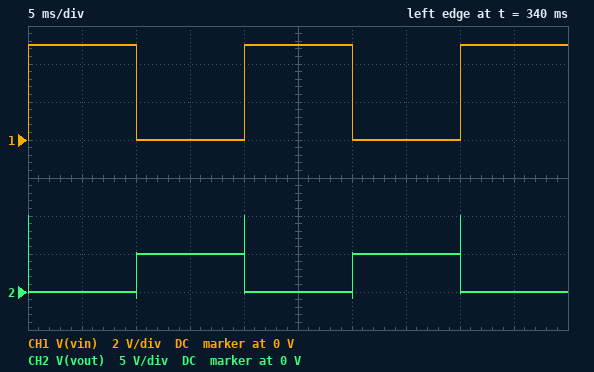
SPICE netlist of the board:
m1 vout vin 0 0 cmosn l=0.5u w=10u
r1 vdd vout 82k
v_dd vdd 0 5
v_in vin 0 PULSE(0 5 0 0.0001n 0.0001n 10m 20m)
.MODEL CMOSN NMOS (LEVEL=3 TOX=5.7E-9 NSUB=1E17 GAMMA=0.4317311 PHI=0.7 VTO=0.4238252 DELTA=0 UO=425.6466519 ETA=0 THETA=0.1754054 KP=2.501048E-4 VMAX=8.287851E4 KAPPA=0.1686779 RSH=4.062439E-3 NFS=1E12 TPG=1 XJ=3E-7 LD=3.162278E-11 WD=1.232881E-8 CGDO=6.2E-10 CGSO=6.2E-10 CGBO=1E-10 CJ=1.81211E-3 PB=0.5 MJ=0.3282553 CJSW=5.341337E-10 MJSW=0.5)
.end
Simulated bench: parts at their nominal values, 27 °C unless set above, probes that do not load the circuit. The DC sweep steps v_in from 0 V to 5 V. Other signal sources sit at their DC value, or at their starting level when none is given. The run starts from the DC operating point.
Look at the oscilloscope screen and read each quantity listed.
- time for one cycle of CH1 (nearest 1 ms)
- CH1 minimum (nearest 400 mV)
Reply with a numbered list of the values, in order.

1. 20 ms
2. 0 V
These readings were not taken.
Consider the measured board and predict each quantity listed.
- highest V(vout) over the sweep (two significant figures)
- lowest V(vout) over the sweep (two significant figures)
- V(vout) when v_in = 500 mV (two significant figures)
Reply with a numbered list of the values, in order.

1. 5.0 V
2. 4.8 mV
3. 1.5 V
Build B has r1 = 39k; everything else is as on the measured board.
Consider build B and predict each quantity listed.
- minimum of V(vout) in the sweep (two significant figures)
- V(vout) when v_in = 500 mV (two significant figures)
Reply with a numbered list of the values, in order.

1. 10 mV
2. 3.2 V
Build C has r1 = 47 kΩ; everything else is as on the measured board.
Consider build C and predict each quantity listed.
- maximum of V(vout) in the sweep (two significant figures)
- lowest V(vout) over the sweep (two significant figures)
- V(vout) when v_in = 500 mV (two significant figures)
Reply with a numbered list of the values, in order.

1. 5.0 V
2. 8.4 mV
3. 2.9 V
